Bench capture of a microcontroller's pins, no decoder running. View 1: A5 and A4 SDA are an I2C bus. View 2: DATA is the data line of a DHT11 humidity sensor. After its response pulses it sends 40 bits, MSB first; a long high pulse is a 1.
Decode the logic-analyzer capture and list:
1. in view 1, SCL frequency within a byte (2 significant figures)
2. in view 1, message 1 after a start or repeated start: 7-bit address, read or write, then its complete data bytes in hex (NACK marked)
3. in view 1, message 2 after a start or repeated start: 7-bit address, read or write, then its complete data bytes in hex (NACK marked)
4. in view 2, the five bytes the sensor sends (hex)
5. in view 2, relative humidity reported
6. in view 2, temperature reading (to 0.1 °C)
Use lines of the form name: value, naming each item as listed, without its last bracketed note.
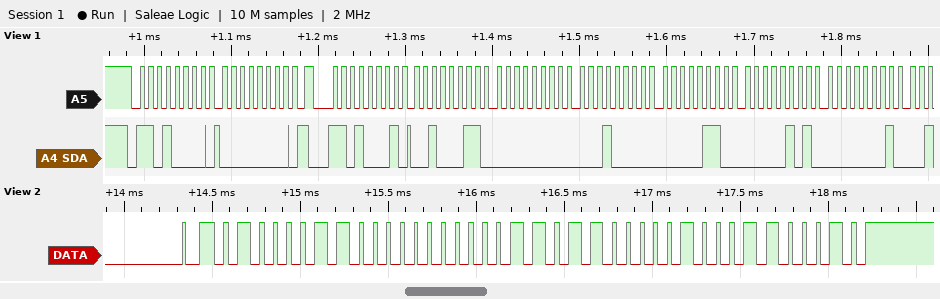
in view 1, SCL frequency within a byte: 100 kHz
in view 1, message 1 after a start or repeated start: 7-bit address, read or write, then its complete data bytes in hex: 0x68 write: 00
in view 1, message 2 after a start or repeated start: 7-bit address, read or write, then its complete data bytes in hex: 0x68 read: 23 00 10 06 05 01
in view 2, the five bytes the sensor sends: 43 00 1B 04 62
in view 2, relative humidity reported: 67 %
in view 2, temperature reading: 27.4 °C
